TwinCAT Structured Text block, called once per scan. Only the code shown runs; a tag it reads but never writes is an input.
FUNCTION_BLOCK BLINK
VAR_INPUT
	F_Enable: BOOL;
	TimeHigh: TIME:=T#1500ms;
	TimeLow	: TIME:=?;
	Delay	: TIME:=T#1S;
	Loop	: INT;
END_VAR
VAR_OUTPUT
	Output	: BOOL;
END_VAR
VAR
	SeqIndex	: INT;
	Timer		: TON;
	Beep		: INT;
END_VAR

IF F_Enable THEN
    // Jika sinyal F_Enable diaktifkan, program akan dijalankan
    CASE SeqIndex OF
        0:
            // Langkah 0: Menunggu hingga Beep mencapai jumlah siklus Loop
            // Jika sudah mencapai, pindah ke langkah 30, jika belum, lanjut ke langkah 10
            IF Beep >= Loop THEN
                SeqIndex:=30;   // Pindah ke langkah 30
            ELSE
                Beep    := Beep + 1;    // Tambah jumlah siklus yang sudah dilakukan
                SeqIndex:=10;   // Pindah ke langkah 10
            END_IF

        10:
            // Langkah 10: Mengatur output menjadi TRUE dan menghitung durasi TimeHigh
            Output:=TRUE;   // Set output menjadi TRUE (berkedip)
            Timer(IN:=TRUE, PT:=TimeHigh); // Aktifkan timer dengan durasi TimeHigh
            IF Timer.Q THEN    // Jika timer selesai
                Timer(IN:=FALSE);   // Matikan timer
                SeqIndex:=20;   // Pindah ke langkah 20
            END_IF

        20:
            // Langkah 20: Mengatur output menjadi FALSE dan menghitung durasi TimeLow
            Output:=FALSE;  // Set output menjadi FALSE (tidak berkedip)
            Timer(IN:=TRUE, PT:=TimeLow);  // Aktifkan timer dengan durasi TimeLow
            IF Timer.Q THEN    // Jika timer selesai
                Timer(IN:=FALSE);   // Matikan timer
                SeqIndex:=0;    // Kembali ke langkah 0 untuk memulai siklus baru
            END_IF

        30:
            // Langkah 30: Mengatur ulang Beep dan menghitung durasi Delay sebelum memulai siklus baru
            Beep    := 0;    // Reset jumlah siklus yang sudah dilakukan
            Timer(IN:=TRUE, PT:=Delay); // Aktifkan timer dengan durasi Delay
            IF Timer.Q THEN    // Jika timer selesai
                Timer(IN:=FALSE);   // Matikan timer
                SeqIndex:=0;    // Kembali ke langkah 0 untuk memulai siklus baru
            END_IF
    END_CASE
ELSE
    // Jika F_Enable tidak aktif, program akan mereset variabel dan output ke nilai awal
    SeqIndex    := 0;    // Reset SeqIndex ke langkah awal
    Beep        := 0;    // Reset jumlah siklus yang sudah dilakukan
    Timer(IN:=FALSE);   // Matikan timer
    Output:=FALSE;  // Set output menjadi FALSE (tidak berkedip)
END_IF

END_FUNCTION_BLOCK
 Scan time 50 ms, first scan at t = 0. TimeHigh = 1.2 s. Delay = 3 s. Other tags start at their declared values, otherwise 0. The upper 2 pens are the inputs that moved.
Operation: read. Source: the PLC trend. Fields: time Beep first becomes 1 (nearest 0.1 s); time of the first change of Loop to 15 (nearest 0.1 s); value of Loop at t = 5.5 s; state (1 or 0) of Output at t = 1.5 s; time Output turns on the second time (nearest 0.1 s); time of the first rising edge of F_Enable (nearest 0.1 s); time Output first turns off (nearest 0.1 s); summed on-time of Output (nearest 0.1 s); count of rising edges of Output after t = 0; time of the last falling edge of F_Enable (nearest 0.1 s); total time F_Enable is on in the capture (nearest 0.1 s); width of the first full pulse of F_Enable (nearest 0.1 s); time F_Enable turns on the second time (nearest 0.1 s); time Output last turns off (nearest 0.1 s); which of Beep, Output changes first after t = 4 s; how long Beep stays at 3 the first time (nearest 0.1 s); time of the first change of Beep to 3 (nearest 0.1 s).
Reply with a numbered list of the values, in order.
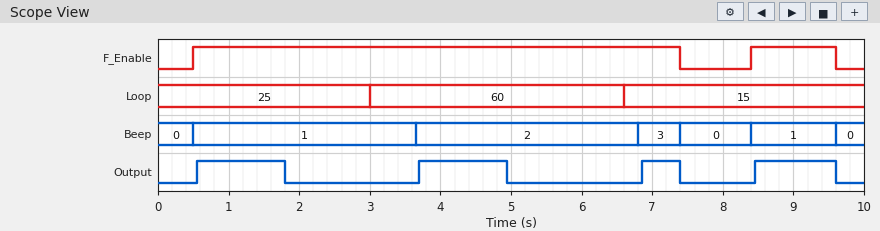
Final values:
1. 0.5 s
2. 6.6 s
3. 60
4. 1
5. 3.7 s
6. 0.5 s
7. 1.8 s
8. 4.2 s
9. 4
10. 9.6 s
11. 8.1 s
12. 6.9 s
13. 8.4 s
14. 9.6 s
15. Output
16. 0.6 s
17. 6.8 s
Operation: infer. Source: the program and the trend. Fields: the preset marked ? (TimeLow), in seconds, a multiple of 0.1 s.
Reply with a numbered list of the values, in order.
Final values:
1. 1.8 s
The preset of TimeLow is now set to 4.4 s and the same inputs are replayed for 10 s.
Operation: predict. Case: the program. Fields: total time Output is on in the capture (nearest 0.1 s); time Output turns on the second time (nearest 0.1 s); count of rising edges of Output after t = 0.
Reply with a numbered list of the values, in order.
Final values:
1. 3.5 s
2. 6.3 s
3. 3
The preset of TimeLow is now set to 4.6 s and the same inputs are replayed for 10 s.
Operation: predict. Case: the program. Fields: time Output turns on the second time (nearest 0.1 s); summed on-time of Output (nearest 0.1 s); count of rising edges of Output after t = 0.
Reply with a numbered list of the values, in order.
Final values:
1. 6.5 s
2. 3.3 s
3. 3
